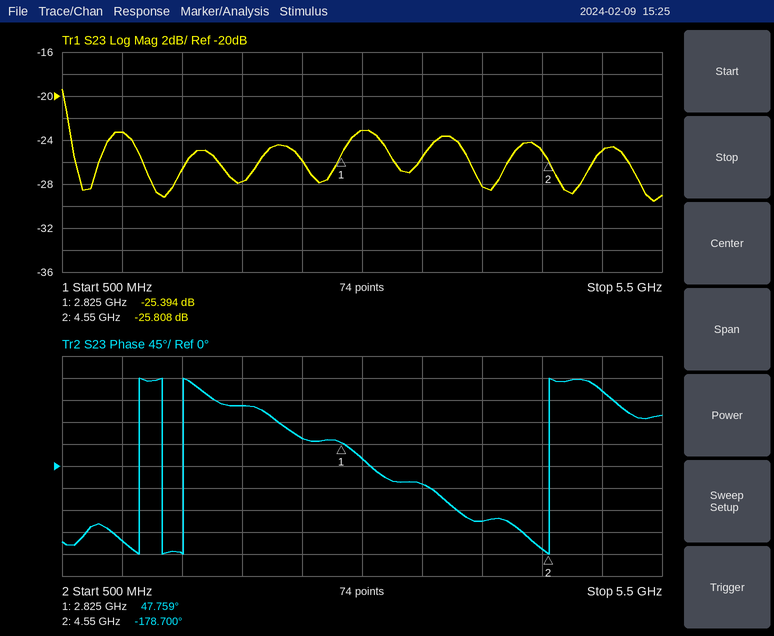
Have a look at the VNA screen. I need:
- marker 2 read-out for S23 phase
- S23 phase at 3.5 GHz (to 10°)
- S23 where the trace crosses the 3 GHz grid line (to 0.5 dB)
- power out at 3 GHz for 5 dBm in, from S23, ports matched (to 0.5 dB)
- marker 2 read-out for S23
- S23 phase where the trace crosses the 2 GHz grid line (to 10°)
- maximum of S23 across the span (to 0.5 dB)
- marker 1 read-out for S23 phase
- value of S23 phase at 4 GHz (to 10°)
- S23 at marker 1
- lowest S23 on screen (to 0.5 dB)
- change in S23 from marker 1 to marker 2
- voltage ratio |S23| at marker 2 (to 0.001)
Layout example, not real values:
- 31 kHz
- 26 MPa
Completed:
- -178.700°
- -40°
- -23.0 dB
- -18.0 dBm
- -25.808 dB
- 120°
- -19.5 dB
- 47.759°
- -110°
- -25.394 dB
- -29.5 dB
- -0.414 dB
- 0.051
